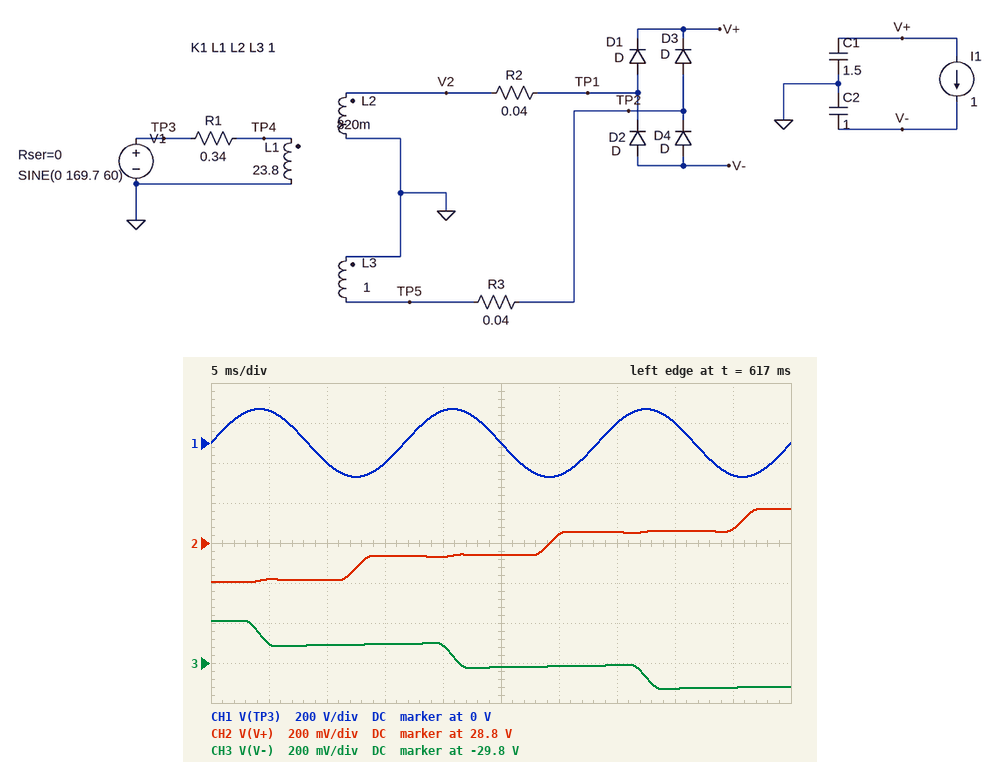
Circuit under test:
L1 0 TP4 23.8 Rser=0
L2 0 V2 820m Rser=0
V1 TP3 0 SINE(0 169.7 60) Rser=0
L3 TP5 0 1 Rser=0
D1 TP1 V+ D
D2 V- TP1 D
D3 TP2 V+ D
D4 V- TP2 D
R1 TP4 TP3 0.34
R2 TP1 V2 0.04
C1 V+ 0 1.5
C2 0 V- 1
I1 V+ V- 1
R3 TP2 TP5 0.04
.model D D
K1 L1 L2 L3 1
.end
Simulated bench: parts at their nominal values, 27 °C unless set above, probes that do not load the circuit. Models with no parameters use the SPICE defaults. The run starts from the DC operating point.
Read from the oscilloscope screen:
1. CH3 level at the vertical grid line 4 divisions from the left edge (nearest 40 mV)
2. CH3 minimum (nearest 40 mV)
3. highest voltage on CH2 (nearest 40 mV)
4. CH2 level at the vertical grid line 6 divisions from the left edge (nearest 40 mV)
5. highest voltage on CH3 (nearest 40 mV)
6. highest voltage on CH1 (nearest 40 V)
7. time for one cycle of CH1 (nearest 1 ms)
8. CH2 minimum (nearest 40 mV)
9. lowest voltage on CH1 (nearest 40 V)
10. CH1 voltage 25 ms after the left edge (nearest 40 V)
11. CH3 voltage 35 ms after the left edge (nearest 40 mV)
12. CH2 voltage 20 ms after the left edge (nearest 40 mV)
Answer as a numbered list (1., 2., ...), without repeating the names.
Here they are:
1. -29.72 V
2. -29.92 V
3. 28.96 V
4. 28.84 V
5. -29.60 V
6. 160 V
7. 17 ms
8. 28.60 V
9. -160 V
10. 0 V
11. -29.80 V
12. 28.72 V
